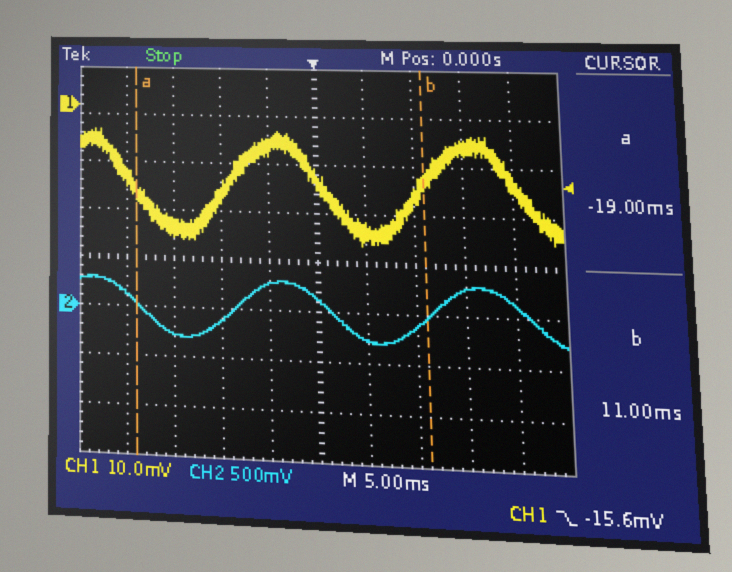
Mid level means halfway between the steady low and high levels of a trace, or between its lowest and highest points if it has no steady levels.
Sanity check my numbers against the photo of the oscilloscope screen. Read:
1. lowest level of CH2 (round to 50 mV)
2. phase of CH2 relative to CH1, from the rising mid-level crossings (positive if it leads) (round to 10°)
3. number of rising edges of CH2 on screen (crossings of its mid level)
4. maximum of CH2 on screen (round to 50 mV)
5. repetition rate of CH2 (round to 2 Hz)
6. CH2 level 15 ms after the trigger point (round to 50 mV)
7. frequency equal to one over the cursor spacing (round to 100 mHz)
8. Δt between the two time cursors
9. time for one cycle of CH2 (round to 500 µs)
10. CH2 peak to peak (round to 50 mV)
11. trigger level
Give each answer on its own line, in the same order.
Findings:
-300 mV
-10°
2
300 mV
50 Hz
250 mV
33.3 Hz
30.0 ms
20.0 ms
600 mV
-15.6 mV
